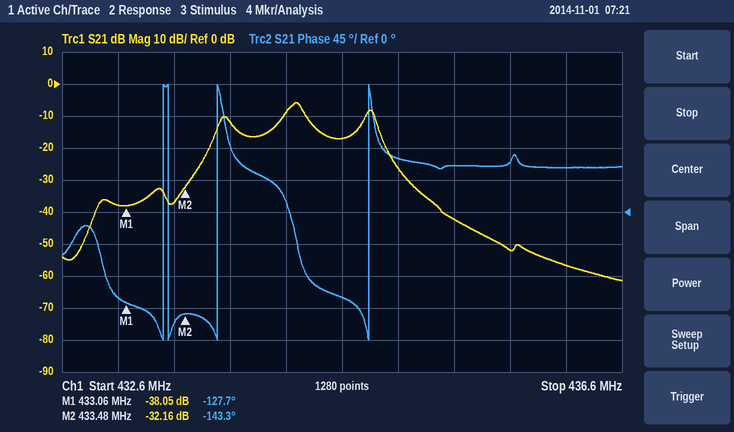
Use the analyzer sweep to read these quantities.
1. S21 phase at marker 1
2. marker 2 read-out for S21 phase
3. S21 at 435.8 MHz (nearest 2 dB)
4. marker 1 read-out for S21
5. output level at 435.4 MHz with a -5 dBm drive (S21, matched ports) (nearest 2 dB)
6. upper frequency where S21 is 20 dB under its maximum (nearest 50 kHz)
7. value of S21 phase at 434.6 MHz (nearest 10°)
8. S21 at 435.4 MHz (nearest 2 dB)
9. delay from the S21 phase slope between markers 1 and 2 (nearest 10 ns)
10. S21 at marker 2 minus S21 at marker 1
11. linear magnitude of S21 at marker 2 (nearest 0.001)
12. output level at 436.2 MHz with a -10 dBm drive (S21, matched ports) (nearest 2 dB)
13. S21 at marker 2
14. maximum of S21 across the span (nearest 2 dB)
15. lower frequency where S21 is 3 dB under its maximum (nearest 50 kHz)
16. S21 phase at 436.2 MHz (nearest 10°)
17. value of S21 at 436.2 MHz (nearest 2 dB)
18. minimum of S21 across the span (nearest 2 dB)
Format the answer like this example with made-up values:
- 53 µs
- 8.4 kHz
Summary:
- -127.7°
- -143.3°
- -52 dB
- -38.05 dB
- -48 dBm
- 435.00 MHz
- -120°
- -42 dB
- 100 ns
- 5.89 dB
- 0.025
- -66 dBm
- -32.16 dB
- -6 dB
- 434.20 MHz
- 60°
- -56 dB
- -62 dB
